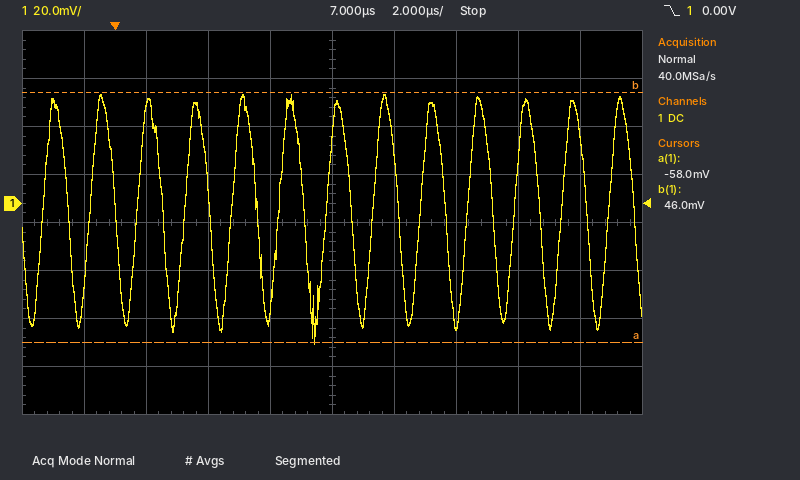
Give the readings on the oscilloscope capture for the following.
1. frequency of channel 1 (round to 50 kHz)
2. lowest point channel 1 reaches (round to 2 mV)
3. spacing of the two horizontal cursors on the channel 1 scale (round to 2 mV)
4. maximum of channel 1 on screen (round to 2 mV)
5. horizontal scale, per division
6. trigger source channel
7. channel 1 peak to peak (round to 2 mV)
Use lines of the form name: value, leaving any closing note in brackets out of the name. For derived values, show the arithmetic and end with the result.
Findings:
frequency of channel 1: 650 kHz
lowest point channel 1 reaches: -58 mV
spacing of the two horizontal cursors on the channel 1 scale: 104 mV
maximum of channel 1 on screen: 46 mV
horizontal scale, per division: 2 µs
trigger source channel: channel 1
channel 1 peak to peak: 46 mV − (-58 mV) = 104 mV
